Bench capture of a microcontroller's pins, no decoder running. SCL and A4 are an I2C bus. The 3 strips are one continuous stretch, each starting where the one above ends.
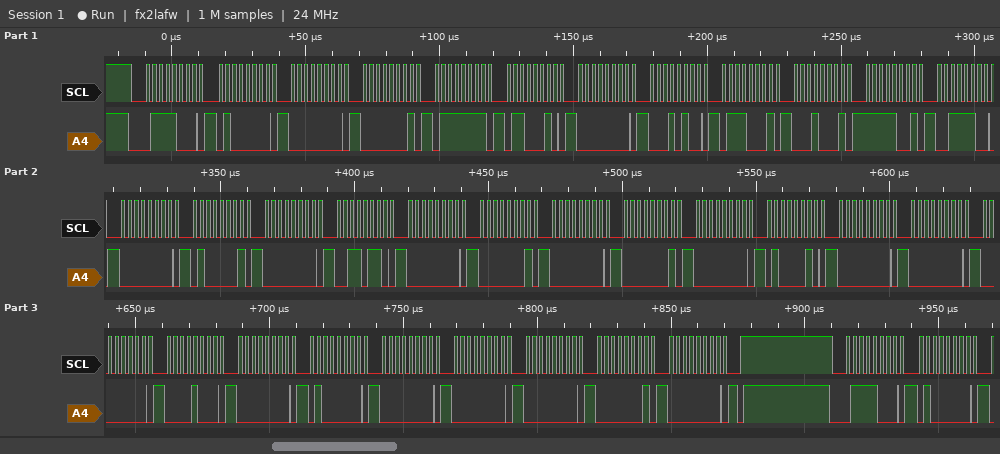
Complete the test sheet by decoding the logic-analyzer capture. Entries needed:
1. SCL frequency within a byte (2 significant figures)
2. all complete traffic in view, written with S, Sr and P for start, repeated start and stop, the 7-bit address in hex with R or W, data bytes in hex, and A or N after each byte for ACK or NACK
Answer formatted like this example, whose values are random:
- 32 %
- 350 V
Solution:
- 400 kHz
- S 3CW A 40 A 00 A 01 A 7F A 62 A 00 A 14 A 71 A 11 A F9 A 3C A 00 A 41 A 00 A 36 A 00 A 01 A 00 A 01 A 00 A 42 A 00 A 00 A 00 A 08 A 00 A 40 A 00 A 00 A 00 A 01 A 00 A P S 3CW A 40 A
